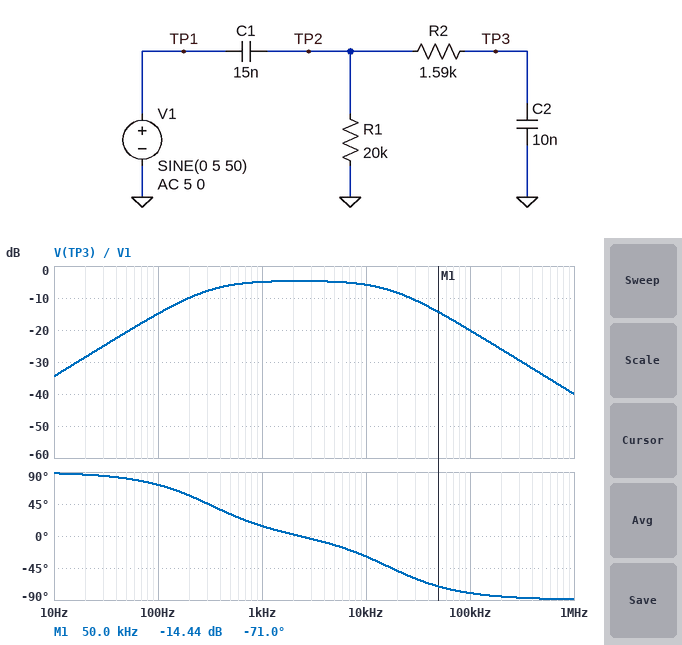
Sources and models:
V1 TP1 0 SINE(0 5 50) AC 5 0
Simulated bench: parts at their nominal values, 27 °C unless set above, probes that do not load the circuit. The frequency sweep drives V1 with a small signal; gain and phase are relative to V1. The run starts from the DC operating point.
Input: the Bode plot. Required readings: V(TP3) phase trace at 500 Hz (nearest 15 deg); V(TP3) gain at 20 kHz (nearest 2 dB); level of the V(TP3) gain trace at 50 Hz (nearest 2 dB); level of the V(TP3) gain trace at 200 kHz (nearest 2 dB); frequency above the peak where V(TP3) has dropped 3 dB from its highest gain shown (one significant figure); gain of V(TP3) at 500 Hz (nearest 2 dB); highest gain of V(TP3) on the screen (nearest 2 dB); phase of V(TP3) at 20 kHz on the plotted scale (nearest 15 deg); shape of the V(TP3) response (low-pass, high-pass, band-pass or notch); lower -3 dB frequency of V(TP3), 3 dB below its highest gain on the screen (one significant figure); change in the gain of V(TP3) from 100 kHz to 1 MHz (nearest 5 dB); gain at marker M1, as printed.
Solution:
30 deg
-8 dB
-20 dB
-26 dB
20 kHz
-6 dB
-4 dB
-45 deg
band-pass
300 Hz
-20 dB
-14.44 dB
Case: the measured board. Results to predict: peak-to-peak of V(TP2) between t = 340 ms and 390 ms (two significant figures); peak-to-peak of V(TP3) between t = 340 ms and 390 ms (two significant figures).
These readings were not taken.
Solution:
930 mV
930 mV
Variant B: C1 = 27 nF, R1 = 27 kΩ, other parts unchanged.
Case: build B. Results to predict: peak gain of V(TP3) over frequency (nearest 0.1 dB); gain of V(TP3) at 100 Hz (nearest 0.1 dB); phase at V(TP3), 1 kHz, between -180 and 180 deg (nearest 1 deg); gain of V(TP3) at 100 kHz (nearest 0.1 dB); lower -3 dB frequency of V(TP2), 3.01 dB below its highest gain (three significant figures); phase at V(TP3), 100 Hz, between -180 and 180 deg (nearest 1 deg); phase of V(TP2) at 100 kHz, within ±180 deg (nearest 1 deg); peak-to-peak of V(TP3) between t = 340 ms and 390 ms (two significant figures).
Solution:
-2.9 dB
-8.2 dB
5 deg
-20.1 dB
659 Hz
57 deg
2 deg
2.2 V
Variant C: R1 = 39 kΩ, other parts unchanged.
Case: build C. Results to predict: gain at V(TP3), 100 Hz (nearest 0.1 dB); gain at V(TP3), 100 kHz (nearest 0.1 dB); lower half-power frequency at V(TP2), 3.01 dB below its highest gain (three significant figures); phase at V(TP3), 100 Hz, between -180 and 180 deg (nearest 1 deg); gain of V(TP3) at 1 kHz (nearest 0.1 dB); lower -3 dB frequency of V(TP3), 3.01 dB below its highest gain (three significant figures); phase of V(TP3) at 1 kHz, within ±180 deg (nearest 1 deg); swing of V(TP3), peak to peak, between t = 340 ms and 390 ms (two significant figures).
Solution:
-10.1 dB
-20.1 dB
9.04 kHz
58 deg
-4.6 dB
159 Hz
6 deg
1.8 V
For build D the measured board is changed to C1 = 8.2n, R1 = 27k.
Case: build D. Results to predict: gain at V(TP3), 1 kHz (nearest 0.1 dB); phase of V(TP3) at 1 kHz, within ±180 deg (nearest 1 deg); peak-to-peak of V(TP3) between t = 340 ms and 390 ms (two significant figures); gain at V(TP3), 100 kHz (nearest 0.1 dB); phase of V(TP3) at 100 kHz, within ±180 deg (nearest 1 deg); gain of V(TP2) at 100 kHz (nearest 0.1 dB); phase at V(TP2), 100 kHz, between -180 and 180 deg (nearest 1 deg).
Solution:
-7.5 dB
15 deg
690 mV
-20.2 dB
-77 deg
-0.2 dB
7 deg
